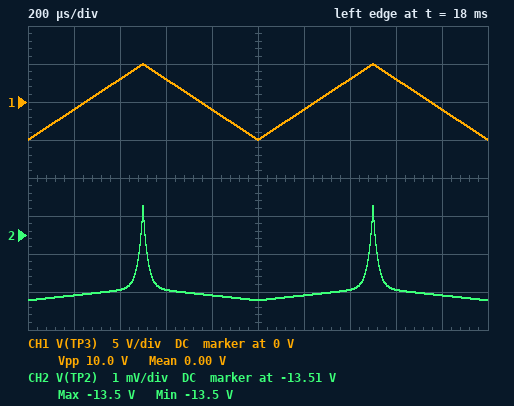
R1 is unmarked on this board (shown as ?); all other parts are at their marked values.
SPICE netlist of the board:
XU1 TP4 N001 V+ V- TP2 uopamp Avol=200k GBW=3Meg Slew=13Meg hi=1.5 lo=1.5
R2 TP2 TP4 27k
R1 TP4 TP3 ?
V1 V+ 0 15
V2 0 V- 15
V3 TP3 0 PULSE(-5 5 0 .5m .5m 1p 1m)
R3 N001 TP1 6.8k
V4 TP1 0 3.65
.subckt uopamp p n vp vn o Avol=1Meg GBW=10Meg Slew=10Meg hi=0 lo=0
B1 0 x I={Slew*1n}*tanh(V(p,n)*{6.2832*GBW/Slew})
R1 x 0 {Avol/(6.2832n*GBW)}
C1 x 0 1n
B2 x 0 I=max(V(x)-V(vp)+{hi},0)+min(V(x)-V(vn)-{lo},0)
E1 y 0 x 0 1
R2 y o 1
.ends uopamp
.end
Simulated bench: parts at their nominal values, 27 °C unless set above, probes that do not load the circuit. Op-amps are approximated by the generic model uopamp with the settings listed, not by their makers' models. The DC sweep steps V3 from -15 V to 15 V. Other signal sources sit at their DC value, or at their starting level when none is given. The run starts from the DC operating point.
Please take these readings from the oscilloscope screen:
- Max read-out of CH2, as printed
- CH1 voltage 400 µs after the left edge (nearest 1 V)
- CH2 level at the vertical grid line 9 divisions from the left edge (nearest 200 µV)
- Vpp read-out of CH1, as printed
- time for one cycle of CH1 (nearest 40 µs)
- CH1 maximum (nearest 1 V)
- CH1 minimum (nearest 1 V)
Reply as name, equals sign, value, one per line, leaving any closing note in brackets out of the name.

Max read-out of CH2, as printed = -13.5 V
CH1 voltage 400 µs after the left edge = 3 V
CH2 level at the vertical grid line 9 divisions from the left edge = -13.5126 V
Vpp read-out of CH1, as printed = 10.0 V
time for one cycle of CH1 = 1.00 ms
CH1 maximum = 5 V
CH1 minimum = -5 V
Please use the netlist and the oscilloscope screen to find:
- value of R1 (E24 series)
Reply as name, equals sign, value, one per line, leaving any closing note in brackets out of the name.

value of R1 = 3.6 kΩ
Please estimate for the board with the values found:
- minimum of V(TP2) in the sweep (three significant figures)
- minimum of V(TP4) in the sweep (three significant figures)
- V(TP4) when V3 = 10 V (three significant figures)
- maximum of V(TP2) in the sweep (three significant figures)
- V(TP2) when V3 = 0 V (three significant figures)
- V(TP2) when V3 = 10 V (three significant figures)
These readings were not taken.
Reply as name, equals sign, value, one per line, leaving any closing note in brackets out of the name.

minimum of V(TP2) in the sweep = -13.5 V
minimum of V(TP4) in the sweep = -14.8 V
V(TP4) when V3 = 10 V = 10.4 V
maximum of V(TP2) in the sweep = 13.5 V
V(TP2) when V3 = 0 V = -13.5 V
V(TP2) when V3 = 10 V = 13.5 V
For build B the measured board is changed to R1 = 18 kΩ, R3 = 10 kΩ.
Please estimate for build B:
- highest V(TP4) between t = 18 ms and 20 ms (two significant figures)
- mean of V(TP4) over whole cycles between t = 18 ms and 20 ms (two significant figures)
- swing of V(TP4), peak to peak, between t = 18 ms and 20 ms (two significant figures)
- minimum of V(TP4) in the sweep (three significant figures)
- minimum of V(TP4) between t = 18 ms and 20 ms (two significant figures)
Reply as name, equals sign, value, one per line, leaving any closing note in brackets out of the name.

highest V(TP4) between t = 18 ms and 20 ms = -2.4 V
mean of V(TP4) over whole cycles between t = 18 ms and 20 ms = -5.4 V
swing of V(TP4), peak to peak, between t = 18 ms and 20 ms = 6.0 V
minimum of V(TP4) in the sweep = -14.4 V
minimum of V(TP4) between t = 18 ms and 20 ms = -8.4 V
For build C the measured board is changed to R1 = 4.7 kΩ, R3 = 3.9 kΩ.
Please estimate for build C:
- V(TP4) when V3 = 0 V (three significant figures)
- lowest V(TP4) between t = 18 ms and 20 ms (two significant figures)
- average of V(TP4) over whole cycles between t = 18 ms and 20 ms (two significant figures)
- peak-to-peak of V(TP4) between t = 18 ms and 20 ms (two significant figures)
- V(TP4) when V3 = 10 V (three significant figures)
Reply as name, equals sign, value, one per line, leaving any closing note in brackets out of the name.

V(TP4) when V3 = 0 V = -2.00 V
lowest V(TP4) between t = 18 ms and 20 ms = -6.3 V
average of V(TP4) over whole cycles between t = 18 ms and 20 ms = -2.0 V
peak-to-peak of V(TP4) between t = 18 ms and 20 ms = 8.5 V
V(TP4) when V3 = 10 V = 10.5 V
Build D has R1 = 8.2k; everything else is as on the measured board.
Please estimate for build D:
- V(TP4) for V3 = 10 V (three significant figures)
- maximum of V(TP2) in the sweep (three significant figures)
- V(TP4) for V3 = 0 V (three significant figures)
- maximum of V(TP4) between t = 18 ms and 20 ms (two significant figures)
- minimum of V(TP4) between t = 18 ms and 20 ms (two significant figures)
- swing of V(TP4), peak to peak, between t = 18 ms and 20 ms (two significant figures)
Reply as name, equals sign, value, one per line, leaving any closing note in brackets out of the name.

V(TP4) for V3 = 10 V = 10.8 V
maximum of V(TP2) in the sweep = 13.5 V
V(TP4) for V3 = 0 V = -3.15 V
maximum of V(TP4) between t = 18 ms and 20 ms = 690 mV
minimum of V(TP4) between t = 18 ms and 20 ms = -7.0 V
swing of V(TP4), peak to peak, between t = 18 ms and 20 ms = 7.7 V
